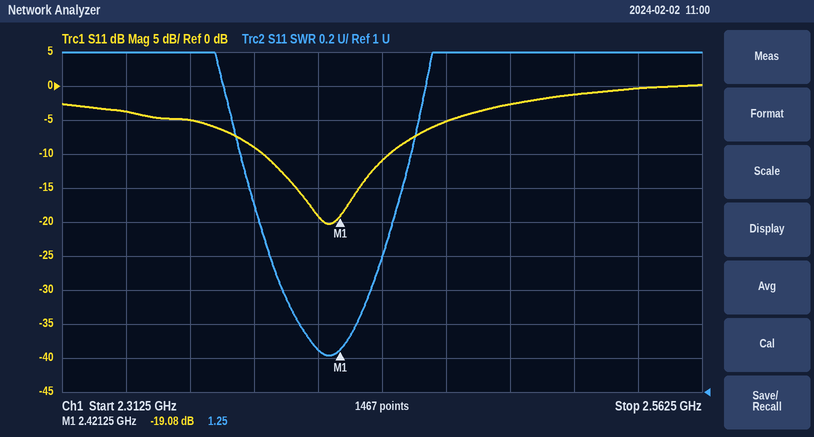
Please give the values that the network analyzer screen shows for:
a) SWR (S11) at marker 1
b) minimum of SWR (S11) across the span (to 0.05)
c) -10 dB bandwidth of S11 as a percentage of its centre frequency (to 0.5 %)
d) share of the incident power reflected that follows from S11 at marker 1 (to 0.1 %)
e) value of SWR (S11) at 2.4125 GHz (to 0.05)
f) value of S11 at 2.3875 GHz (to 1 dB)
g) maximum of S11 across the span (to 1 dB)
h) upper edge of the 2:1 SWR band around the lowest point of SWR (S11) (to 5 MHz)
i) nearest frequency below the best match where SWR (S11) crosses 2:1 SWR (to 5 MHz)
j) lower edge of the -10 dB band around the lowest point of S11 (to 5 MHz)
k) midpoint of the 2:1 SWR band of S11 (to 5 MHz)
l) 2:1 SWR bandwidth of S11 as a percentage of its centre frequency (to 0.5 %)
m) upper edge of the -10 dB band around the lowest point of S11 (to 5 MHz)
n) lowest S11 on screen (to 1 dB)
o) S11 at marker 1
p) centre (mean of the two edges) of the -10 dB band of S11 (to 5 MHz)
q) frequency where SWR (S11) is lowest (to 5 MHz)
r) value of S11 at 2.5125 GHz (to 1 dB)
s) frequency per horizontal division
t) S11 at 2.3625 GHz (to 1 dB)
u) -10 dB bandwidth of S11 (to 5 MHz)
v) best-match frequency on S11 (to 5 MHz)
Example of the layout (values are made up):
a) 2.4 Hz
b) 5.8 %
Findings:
a) 1.25
b) 1.20
c) 2.0 %
d) 1.2 %
e) 1.25
f) -9 dB
g) 0 dB
h) 2.440 GHz
i) 2.390 GHz
j) 2.390 GHz
k) 2.415 GHz
l) 2.0 %
m) 2.440 GHz
n) -20 dB
o) -19.08 dB
p) 2.415 GHz
q) 2.415 GHz
r) -1 dB
s) 25 MHz
t) -5 dB
u) 50 MHz
v) 2.415 GHz
